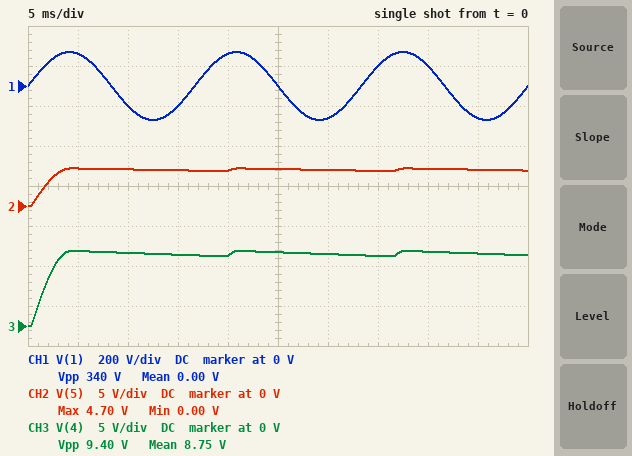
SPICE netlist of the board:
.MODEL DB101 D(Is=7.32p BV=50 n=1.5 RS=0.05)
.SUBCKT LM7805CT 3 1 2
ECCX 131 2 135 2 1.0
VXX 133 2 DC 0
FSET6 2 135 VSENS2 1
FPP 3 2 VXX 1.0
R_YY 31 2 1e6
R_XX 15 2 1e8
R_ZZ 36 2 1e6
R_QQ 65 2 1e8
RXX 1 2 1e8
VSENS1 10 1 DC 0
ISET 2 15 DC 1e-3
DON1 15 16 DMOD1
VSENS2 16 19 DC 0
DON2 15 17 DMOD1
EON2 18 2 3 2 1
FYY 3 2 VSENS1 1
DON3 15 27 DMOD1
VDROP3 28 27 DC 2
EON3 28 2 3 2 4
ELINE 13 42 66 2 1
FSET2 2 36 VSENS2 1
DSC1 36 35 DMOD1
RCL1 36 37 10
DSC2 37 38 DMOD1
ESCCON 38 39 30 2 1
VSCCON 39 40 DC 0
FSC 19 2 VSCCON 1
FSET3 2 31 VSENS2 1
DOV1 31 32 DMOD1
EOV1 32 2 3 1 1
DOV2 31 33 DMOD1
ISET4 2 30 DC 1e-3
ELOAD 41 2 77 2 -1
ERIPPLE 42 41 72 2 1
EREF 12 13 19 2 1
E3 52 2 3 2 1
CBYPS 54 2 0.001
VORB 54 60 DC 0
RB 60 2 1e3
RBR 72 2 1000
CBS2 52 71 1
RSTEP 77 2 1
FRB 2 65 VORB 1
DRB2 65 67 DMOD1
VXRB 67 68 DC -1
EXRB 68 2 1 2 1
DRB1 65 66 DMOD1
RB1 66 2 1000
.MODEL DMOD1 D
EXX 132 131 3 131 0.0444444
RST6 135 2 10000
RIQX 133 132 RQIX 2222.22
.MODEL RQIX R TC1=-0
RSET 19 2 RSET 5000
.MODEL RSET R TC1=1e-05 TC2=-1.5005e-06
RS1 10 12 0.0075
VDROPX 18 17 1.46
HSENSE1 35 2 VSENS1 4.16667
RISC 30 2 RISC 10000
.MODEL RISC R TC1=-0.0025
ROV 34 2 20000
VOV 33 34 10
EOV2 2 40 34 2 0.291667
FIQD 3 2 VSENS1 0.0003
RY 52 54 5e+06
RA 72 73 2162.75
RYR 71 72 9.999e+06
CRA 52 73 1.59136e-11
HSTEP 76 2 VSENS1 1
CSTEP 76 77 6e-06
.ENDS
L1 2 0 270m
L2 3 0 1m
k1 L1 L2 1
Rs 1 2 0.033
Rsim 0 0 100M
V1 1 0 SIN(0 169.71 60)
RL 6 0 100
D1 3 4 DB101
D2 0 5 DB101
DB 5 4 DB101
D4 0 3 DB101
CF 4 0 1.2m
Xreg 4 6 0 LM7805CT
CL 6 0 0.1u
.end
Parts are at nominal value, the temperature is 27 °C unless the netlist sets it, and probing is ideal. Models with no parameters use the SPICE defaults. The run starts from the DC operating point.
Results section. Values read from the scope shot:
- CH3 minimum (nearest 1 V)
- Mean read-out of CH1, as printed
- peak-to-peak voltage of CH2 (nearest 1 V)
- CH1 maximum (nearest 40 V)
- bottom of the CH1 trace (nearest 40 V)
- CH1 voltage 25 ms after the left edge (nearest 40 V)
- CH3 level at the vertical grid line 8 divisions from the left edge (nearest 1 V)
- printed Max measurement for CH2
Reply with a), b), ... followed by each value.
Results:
a) 0 V
b) 0.00 V
c) 5 V
d) 160 V
e) -160 V
f) 0 V
g) 9 V
h) 4.70 V
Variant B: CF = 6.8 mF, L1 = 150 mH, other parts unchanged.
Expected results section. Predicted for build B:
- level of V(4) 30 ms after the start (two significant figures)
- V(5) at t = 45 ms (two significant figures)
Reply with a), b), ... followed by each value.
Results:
a) 13 V
b) 6.4 V
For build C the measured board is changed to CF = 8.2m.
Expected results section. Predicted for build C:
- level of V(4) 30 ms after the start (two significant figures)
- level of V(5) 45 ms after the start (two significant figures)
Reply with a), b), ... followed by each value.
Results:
a) 9.2 V
b) 4.6 V
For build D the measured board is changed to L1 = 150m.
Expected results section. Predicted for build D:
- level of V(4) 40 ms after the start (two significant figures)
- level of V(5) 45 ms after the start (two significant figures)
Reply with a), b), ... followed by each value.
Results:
a) 13 V
b) 6.3 V
